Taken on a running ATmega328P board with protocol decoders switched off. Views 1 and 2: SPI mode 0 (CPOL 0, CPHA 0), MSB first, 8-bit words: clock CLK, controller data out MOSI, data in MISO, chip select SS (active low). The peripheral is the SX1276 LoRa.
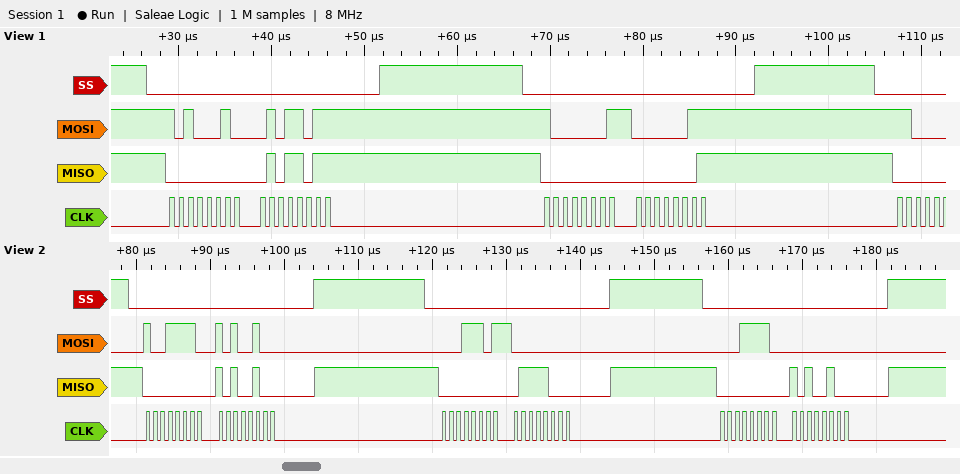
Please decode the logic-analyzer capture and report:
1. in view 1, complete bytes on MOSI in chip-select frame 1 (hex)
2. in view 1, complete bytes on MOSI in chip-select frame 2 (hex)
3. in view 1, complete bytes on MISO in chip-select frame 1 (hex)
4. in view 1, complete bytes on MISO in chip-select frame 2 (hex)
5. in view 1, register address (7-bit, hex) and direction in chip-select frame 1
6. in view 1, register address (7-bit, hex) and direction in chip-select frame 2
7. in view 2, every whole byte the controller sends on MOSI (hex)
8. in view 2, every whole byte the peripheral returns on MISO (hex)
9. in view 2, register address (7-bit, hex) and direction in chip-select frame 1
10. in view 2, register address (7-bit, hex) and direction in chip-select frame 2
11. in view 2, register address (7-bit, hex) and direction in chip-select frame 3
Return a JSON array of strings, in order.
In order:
["0xA2 0x5B", "0x81 0x03", "0x00 0x5B", "0x00 0x01", "0x22 write", "0x01 write", "0x9E 0xA4 0x1D 0x00 0x1E 0x00", "0x00 0xA4 0x00 0x78 0x00 0xA4", "0x1E write", "0x1D read", "0x1E read"]
